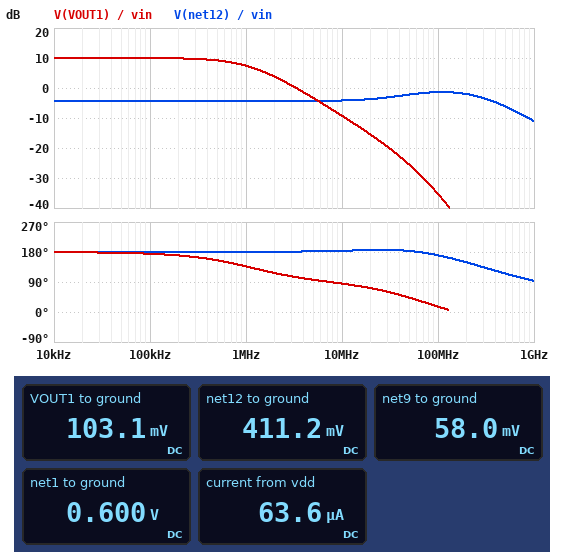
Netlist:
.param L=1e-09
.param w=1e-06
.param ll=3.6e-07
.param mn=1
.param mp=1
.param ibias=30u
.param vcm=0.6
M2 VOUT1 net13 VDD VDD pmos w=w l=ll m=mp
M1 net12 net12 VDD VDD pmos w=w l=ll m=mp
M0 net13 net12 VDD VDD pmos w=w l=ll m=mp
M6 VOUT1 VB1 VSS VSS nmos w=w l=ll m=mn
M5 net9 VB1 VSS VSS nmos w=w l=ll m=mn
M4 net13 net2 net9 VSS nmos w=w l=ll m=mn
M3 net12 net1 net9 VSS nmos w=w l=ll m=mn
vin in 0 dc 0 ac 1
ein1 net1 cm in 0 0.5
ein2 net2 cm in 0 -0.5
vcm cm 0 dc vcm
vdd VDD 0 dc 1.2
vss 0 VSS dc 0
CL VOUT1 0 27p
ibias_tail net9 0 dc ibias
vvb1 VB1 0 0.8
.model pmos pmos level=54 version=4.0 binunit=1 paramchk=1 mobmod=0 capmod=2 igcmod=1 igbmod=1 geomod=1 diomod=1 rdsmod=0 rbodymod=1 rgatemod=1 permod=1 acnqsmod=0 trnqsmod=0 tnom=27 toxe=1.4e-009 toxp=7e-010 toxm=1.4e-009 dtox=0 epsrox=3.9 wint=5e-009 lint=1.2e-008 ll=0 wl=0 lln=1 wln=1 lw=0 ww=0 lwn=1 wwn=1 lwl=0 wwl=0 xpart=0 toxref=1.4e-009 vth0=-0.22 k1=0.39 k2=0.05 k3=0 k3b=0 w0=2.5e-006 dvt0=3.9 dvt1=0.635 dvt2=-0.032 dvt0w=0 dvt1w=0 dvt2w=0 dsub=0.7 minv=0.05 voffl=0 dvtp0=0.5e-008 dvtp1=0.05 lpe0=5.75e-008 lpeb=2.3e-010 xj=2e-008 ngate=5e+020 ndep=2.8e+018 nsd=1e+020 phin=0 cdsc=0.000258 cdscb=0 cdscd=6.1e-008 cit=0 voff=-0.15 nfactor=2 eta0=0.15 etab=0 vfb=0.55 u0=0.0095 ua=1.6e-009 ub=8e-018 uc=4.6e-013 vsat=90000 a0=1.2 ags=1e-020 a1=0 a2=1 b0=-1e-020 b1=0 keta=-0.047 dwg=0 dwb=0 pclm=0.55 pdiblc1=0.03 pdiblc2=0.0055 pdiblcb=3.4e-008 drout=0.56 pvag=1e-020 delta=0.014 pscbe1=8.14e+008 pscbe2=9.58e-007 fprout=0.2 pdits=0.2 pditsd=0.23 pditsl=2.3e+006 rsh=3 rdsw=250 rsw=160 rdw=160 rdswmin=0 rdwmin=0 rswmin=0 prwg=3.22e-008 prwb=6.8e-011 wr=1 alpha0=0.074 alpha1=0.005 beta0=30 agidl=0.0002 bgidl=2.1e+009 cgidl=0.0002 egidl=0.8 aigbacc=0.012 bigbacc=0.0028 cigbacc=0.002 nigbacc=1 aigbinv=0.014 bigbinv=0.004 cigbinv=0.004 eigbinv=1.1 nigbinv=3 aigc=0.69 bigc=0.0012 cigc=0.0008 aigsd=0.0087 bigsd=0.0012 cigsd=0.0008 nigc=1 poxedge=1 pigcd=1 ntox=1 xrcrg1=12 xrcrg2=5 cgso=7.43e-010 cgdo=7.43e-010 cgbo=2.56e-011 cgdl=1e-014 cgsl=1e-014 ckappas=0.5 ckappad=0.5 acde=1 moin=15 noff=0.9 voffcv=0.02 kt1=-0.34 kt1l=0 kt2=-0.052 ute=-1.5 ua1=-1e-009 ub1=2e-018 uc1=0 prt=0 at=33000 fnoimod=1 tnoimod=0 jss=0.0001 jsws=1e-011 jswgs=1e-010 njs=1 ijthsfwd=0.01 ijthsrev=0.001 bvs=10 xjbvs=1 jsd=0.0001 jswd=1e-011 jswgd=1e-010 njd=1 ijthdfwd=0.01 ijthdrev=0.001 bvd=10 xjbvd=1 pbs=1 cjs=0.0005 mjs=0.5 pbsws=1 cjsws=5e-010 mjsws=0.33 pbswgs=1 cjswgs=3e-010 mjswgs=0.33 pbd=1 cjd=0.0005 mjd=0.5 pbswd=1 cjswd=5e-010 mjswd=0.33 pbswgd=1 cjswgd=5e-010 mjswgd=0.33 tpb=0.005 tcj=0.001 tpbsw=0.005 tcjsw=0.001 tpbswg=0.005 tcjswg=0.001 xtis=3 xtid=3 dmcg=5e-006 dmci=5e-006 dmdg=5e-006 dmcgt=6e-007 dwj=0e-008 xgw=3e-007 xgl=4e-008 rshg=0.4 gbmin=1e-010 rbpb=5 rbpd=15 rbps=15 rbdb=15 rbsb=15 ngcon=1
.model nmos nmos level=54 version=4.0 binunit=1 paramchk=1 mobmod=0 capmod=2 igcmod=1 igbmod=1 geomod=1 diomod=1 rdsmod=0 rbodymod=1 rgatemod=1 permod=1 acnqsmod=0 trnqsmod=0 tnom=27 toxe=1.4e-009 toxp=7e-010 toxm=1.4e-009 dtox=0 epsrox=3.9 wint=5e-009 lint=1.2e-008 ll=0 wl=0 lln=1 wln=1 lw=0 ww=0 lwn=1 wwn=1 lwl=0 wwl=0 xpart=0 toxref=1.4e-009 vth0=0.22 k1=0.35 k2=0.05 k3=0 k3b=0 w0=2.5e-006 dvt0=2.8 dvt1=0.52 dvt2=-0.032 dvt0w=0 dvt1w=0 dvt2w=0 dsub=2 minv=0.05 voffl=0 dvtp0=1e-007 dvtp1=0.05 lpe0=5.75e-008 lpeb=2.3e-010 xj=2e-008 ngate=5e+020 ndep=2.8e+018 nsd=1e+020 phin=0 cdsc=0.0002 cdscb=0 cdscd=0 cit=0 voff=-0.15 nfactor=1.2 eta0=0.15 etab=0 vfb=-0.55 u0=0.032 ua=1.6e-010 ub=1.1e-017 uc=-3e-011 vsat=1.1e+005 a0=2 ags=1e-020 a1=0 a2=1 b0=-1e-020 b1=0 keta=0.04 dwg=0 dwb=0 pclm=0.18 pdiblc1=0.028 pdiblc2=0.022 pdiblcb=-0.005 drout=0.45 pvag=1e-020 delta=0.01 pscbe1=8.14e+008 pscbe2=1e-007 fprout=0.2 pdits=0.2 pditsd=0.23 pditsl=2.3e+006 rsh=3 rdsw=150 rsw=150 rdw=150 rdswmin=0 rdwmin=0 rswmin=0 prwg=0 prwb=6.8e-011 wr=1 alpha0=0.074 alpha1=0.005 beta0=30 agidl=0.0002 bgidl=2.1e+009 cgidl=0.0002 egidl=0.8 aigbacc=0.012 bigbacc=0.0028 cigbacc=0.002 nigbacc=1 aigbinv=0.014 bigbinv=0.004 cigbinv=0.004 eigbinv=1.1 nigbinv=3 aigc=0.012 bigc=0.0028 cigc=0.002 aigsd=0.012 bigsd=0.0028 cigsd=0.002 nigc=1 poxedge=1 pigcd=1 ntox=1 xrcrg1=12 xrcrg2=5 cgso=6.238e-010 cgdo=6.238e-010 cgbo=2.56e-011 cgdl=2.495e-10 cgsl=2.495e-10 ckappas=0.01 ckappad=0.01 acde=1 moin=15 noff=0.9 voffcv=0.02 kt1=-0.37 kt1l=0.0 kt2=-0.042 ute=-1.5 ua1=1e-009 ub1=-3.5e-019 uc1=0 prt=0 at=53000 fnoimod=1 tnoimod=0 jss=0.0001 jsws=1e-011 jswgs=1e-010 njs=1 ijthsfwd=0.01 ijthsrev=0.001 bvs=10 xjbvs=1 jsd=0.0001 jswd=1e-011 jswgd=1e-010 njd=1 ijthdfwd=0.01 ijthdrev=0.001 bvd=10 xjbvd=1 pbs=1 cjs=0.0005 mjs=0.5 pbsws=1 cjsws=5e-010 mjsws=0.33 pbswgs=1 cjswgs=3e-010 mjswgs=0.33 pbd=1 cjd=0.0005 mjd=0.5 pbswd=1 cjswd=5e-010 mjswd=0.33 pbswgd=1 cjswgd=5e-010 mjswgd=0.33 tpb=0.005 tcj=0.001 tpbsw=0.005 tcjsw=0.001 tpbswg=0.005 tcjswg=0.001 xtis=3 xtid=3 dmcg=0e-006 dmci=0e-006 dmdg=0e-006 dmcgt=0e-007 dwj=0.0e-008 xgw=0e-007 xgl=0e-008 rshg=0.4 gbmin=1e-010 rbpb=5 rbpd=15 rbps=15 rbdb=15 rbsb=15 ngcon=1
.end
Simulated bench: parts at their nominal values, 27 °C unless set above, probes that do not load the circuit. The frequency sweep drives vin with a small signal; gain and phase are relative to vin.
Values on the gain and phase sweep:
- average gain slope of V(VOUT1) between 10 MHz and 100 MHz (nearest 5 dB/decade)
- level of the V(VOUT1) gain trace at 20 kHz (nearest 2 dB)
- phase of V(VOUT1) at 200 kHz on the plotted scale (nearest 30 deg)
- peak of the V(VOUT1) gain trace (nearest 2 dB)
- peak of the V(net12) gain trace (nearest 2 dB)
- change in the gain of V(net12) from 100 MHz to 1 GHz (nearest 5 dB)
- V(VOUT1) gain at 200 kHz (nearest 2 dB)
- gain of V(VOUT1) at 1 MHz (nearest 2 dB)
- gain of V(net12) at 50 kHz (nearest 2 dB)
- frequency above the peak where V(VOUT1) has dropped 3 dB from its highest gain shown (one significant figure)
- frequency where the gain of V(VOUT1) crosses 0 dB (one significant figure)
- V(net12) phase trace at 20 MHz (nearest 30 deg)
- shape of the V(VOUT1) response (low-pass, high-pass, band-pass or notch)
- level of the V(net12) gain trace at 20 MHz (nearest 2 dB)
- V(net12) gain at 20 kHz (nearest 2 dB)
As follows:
-25 dB/decade
10 dB
180 deg
10 dB
-2 dB
-10 dB
10 dB
8 dB
-4 dB
1 MHz
3 MHz
180 deg
low-pass
-4 dB
-4 dB
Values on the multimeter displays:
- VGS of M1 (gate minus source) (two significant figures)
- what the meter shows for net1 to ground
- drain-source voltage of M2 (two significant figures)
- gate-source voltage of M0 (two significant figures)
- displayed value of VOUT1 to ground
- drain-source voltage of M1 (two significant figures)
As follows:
-790 mV
0.600 V
-1.1 V
-790 mV
103.1 mV
-790 mV
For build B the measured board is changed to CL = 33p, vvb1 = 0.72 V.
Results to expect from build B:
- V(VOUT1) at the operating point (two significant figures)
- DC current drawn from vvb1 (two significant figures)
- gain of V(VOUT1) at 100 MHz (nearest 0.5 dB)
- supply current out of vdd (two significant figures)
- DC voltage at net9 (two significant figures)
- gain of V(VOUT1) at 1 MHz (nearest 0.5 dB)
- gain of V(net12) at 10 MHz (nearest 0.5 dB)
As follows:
110 mV
2.2 µA
-37.0 dB
63 µA
59 mV
7.0 dB
-4.5 dB
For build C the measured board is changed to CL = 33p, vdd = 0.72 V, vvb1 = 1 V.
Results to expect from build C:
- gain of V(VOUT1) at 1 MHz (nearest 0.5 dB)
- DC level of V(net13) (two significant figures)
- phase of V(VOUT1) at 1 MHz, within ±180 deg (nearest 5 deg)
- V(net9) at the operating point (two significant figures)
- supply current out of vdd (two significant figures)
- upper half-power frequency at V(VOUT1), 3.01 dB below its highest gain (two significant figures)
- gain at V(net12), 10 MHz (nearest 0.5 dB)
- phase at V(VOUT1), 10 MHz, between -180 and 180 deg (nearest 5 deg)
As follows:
-34.5 dB
82 mV
140 deg
3.7 mV
41 µA
1.1 MHz
-26.0 dB
95 deg
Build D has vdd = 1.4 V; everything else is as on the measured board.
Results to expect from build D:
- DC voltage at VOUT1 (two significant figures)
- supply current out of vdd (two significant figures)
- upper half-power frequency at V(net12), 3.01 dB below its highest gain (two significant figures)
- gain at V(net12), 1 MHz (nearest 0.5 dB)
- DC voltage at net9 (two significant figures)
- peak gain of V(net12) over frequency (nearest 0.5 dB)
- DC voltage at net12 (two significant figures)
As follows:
110 mV
65 µA
360 MHz
-3.5 dB
62 mV
-1.0 dB
600 mV
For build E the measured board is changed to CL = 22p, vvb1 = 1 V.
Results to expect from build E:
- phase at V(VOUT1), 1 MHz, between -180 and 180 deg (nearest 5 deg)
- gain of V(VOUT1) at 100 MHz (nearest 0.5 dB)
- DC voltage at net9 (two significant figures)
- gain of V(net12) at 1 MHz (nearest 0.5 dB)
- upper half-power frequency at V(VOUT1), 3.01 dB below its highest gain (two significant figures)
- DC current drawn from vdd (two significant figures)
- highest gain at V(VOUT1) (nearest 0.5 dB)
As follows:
145 deg
-33.5 dB
59 mV
-4.0 dB
1.6 MHz
63 µA
9.0 dB
